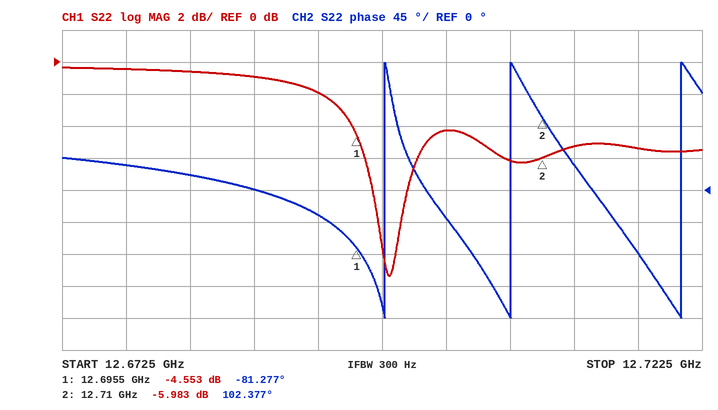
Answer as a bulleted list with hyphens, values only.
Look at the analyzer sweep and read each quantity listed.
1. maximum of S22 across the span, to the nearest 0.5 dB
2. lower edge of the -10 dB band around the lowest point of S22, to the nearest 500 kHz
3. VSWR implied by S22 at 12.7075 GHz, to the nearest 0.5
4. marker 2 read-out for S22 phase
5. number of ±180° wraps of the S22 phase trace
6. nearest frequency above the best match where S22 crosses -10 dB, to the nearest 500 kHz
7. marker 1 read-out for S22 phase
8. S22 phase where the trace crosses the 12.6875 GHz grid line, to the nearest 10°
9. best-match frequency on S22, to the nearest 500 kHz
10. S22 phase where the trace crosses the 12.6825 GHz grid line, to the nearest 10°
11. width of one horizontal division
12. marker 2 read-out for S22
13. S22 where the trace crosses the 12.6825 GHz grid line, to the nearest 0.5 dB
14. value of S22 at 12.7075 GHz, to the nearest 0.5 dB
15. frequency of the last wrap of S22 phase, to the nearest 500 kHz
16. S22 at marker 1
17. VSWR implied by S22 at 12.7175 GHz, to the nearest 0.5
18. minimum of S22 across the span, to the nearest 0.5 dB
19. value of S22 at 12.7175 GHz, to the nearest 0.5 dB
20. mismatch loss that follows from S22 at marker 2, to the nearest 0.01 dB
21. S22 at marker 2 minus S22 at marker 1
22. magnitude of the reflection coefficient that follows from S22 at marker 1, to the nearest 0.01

- -0.5 dB
- 12.6970 GHz
- 3.0
- 102.377°
- 3
- 12.6990 GHz
- -81.277°
- 0°
- 12.6980 GHz
- 20°
- 5 MHz
- -5.983 dB
- -0.5 dB
- -6.0 dB
- 12.7210 GHz
- -4.553 dB
- 3.5
- -13.5 dB
- -5.5 dB
- 1.26 dB
- -1.430 dB
- 0.59
